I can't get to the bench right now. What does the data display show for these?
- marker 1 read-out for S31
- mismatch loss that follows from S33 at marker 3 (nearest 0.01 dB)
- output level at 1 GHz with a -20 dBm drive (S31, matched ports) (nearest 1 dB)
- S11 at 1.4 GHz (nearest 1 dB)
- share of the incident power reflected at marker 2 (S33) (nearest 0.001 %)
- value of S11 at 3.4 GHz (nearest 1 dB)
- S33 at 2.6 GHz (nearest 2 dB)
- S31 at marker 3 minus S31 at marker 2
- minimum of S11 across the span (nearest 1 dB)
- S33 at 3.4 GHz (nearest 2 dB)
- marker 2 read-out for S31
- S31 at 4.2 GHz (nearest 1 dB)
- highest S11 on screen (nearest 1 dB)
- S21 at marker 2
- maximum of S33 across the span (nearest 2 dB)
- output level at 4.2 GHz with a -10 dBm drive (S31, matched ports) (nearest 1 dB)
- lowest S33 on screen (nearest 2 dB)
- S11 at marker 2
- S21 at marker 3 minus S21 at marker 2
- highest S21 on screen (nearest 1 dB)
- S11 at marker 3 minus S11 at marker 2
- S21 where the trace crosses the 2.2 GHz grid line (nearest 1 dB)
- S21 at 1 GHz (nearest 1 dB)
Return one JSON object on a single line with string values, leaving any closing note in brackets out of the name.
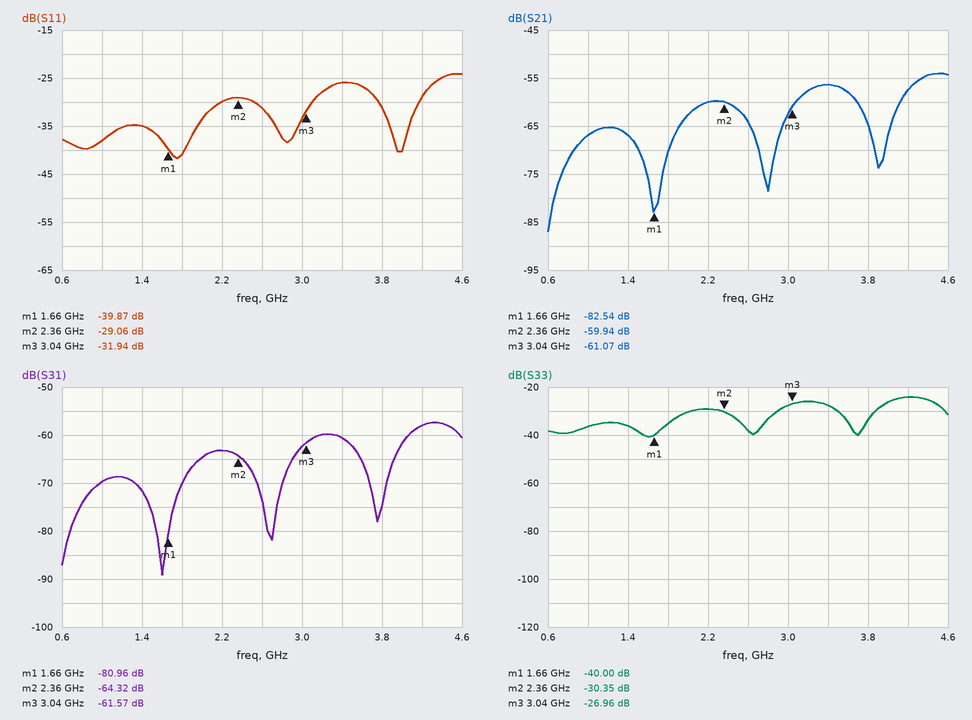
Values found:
{"marker 1 read-out for S31": "-80.96 dB", "mismatch loss that follows from S33 at marker 3": "0.01 dB", "output level at 1 GHz with a -20 dBm drive (S31, matched ports)": "-90 dBm", "S11 at 1.4 GHz": "-35 dB", "share of the incident power reflected at marker 2 (S33)": "0.092 %", "value of S11 at 3.4 GHz": "-26 dB", "S33 at 2.6 GHz": "-38 dB", "S31 at marker 3 minus S31 at marker 2": "2.75 dB", "minimum of S11 across the span": "-42 dB", "S33 at 3.4 GHz": "-28 dB", "marker 2 read-out for S31": "-64.32 dB", "S31 at 4.2 GHz": "-58 dB", "highest S11 on screen": "-24 dB", "S21 at marker 2": "-59.94 dB", "maximum of S33 across the span": "-24 dB", "output level at 4.2 GHz with a -10 dBm drive (S31, matched ports)": "-68 dBm", "lowest S33 on screen": "-40 dB", "S11 at marker 2": "-29.06 dB", "S21 at marker 3 minus S21 at marker 2": "-1.13 dB", "highest S21 on screen": "-54 dB", "S11 at marker 3 minus S11 at marker 2": "-2.88 dB", "S21 where the trace crosses the 2.2 GHz grid line": "-60 dB", "S21 at 1 GHz": "-67 dB"}
